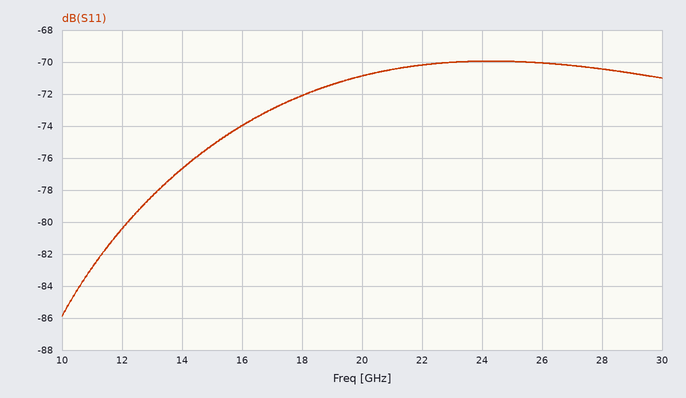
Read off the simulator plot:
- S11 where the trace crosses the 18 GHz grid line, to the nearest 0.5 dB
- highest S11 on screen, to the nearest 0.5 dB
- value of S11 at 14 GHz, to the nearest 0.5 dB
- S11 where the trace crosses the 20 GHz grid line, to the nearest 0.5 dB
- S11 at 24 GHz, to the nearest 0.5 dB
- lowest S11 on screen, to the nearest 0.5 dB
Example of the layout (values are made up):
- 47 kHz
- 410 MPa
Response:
- -72.0 dB
- -70.0 dB
- -76.5 dB
- -71.0 dB
- -70.0 dB
- -86.0 dB
